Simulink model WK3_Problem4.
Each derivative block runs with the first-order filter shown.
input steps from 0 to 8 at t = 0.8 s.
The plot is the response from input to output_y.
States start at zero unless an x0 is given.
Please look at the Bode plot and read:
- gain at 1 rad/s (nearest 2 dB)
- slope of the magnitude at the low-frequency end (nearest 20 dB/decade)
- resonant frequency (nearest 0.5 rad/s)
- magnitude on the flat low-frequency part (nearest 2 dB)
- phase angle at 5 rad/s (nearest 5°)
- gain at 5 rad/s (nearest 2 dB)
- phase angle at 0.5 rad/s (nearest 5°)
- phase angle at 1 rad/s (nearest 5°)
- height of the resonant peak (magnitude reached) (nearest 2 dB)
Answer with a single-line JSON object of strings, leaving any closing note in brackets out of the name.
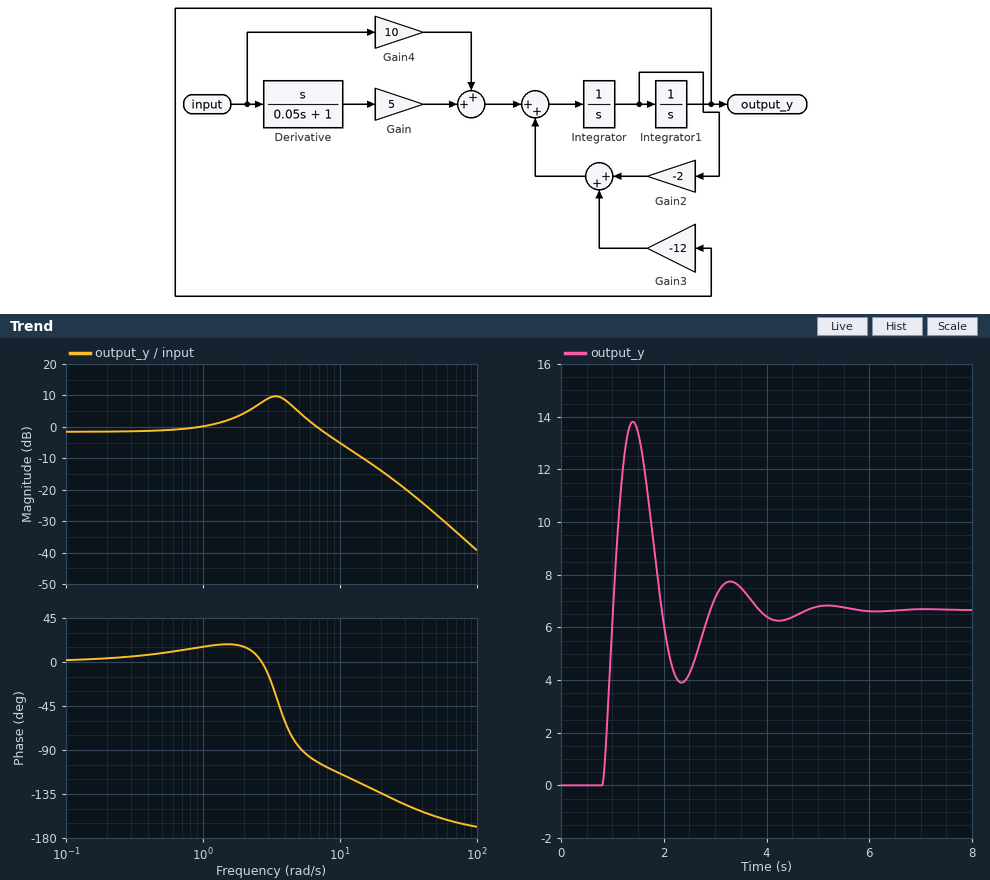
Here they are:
{"gain at 1 rad/s": "0 dB", "slope of the magnitude at the low-frequency end": "0 dB/decade", "resonant frequency": "3.5 rad/s", "magnitude on the flat low-frequency part": "-2 dB", "phase angle at 5 rad/s": "-85°", "gain at 5 rad/s": "4 dB", "phase angle at 0.5 rad/s": "10°", "phase angle at 1 rad/s": "15°", "height of the resonant peak (magnitude reached)": "10 dB"}
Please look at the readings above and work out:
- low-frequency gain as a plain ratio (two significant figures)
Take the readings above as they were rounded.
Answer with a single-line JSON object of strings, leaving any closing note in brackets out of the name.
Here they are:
{"low-frequency gain as a plain ratio": "0.79"}
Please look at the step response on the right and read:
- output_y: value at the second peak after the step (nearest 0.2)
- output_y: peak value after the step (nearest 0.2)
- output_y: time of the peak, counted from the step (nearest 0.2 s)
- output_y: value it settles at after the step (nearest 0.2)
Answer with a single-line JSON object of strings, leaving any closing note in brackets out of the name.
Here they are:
{"output_y: value at the second peak after the step": "7.8", "output_y: peak value after the step": "13.8", "output_y: time of the peak, counted from the step": "0.6 s", "output_y: value it settles at after the step": "6.6"}
